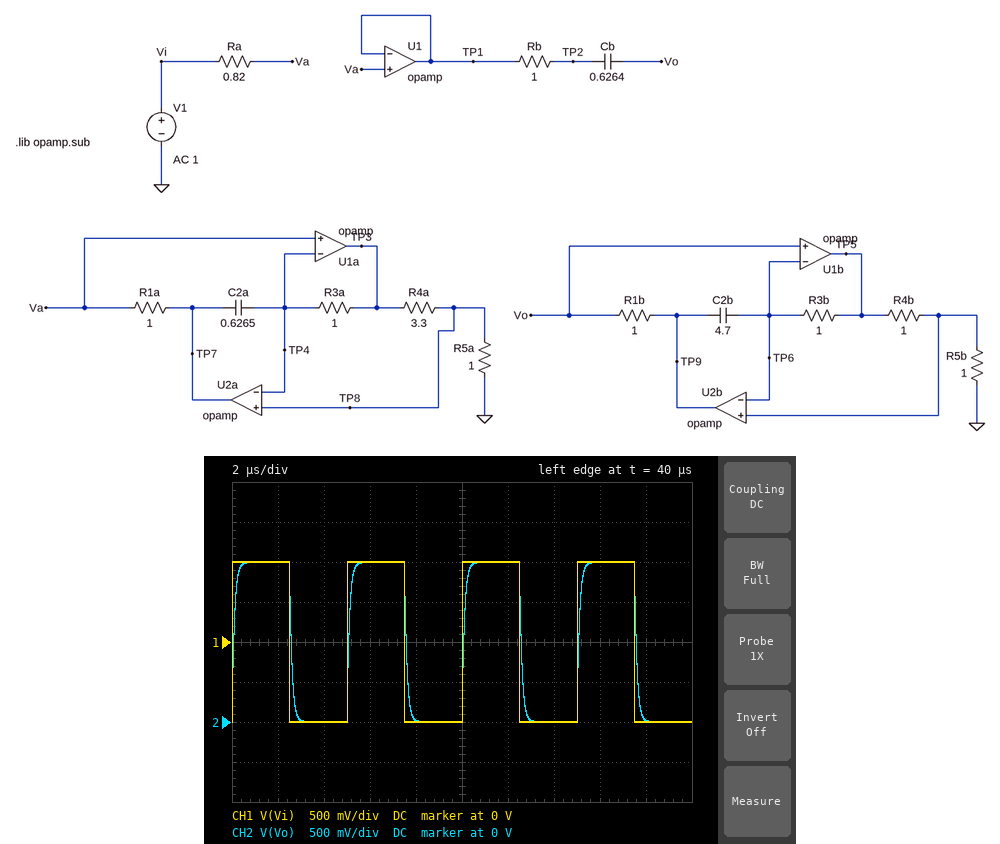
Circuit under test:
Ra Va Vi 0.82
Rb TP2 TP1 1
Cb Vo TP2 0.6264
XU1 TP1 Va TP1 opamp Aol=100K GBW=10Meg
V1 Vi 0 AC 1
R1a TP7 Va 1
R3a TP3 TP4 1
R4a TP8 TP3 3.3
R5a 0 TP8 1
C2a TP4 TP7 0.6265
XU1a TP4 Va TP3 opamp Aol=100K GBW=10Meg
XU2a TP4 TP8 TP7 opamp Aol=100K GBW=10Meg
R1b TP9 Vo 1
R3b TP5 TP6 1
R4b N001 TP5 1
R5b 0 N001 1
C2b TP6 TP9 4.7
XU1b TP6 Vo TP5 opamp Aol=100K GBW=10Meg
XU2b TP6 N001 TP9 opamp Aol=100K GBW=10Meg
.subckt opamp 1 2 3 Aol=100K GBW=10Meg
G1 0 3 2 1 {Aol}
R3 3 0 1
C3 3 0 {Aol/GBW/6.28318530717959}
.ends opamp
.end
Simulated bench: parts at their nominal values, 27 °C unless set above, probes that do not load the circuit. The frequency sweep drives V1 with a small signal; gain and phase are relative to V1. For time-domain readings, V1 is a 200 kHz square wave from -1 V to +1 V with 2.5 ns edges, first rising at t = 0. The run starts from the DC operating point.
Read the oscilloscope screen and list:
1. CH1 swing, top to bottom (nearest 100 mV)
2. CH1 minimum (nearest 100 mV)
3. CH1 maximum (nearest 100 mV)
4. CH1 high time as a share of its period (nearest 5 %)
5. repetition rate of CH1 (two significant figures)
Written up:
2.0 V
-1.0 V
1.0 V
50 %
200 kHz
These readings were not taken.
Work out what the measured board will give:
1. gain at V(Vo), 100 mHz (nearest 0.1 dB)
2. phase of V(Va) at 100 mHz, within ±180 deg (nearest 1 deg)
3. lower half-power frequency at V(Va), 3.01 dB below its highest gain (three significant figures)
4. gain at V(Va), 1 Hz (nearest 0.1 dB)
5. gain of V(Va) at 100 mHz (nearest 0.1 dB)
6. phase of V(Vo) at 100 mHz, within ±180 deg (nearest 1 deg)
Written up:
-8.1 dB
82 deg
687 mHz
-1.7 dB
-16.8 dB
149 deg
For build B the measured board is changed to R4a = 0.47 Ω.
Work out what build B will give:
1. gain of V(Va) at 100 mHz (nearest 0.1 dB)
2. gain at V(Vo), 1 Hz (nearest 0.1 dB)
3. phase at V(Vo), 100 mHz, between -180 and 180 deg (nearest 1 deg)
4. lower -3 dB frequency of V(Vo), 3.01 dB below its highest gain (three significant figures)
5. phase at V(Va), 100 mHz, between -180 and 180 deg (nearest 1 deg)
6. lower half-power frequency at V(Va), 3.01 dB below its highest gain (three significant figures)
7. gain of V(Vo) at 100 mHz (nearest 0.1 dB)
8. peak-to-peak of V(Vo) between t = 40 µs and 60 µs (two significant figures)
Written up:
-2.9 dB
0 dB
112 deg
83.5 mHz
44 deg
97.9 mHz
5.8 dB
2.0 V
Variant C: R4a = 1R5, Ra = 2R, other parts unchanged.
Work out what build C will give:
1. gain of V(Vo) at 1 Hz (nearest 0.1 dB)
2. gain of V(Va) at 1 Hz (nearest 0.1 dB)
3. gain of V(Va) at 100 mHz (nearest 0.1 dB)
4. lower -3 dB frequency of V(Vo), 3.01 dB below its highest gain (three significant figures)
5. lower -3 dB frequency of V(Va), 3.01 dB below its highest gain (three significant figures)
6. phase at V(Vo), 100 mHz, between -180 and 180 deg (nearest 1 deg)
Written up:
-1.9 dB
-2.0 dB
-17.7 dB
740 mHz
762 mHz
150 deg
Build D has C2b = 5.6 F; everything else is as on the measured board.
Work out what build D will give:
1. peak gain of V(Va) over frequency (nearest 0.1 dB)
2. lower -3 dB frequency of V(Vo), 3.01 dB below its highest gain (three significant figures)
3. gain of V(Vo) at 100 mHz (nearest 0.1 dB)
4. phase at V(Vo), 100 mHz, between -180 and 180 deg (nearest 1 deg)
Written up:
0 dB
667 mHz
-8.8 dB
127 deg
